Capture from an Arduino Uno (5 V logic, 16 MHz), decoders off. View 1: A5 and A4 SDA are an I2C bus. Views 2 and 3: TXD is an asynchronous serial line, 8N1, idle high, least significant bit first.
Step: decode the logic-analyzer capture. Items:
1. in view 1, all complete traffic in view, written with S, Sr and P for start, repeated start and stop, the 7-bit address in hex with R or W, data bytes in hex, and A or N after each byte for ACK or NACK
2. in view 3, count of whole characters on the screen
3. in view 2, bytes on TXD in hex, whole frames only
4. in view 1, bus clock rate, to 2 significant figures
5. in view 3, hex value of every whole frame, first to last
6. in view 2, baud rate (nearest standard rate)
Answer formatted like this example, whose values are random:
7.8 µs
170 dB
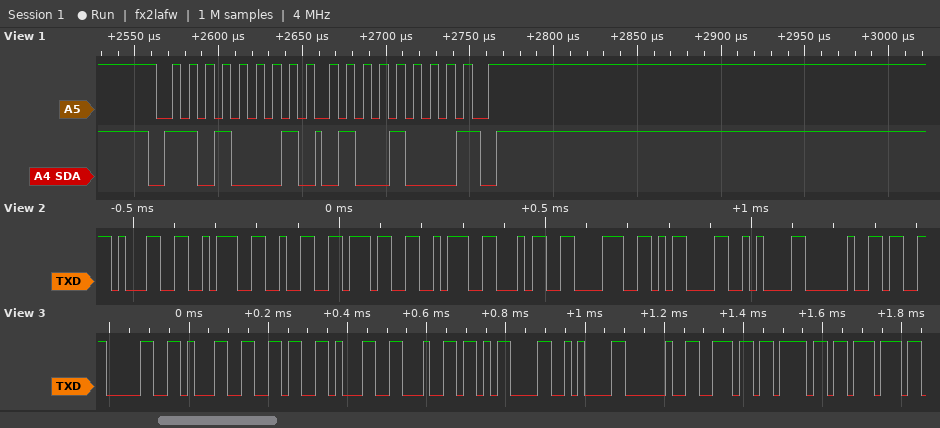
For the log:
S 68R A 48 N P
11
31 3A 32 37 3A 34 38 0D 0A 20
100 kHz
30 31 36 31 64 0D 0A 20 6E 6F 77
57600 baud
